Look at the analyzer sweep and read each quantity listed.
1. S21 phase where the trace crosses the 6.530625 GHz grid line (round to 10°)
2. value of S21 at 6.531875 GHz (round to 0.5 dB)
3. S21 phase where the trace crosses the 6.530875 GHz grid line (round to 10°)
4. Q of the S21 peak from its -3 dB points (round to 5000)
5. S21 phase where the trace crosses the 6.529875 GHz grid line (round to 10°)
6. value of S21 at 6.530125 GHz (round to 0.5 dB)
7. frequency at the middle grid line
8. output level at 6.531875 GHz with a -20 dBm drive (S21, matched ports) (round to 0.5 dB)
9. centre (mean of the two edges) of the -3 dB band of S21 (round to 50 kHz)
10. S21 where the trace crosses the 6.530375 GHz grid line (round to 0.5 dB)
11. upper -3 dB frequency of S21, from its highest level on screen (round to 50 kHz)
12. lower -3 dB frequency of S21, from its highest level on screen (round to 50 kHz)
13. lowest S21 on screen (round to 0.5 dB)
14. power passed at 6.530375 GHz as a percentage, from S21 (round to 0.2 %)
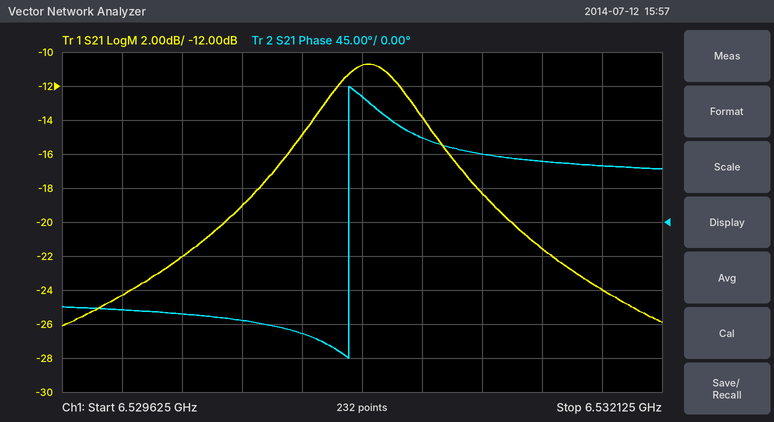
-150°
-24.0 dB
170°
15000
-120°
-22.0 dB
6.530875 GHz
-44.0 dBm
6.53090 GHz
-19.0 dB
6.53110 GHz
6.53070 GHz
-26.0 dB
1.2 %
